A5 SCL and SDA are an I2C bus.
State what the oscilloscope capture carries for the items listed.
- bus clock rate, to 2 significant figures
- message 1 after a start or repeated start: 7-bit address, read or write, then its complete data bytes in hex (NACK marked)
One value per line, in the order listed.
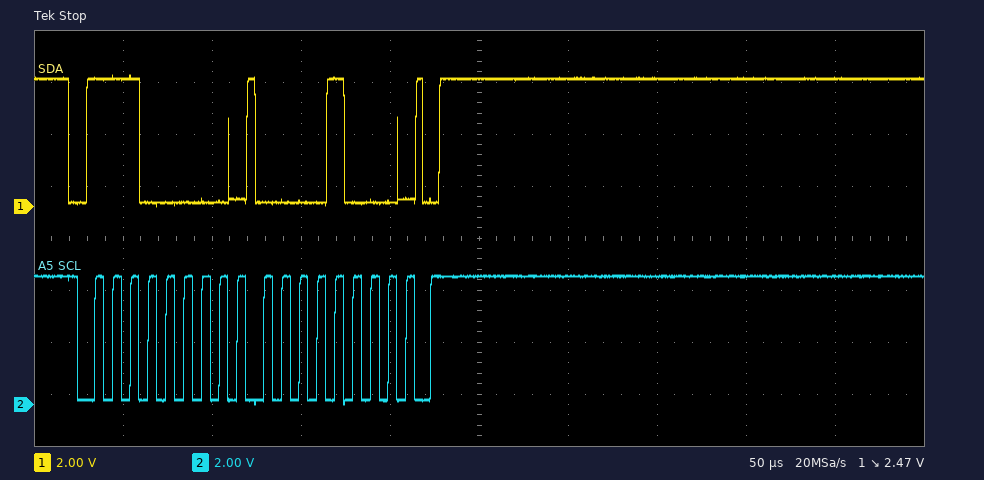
100 kHz
0x70 write: 08
